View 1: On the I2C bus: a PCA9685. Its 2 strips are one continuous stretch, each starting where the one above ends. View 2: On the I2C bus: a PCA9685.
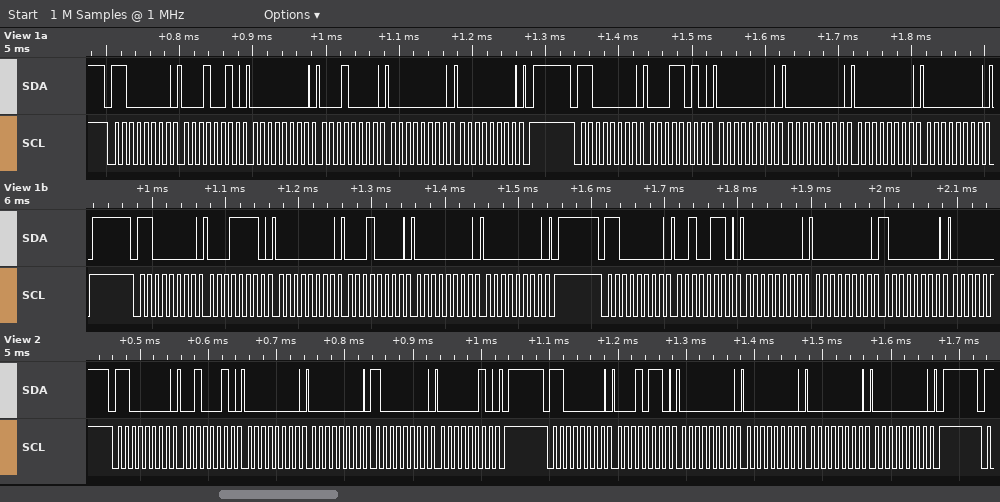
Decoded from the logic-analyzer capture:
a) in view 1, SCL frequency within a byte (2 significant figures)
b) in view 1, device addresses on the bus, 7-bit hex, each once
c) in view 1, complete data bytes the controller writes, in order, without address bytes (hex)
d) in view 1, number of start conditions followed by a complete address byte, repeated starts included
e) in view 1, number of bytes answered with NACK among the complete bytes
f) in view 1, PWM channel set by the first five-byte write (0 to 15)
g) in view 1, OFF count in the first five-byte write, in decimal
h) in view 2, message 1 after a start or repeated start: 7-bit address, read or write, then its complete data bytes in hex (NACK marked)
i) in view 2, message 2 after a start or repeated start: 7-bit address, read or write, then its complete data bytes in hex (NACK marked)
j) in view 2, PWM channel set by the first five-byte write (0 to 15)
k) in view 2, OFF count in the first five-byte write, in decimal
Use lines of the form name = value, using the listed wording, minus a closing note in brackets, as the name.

in view 1, SCL frequency within a byte = 100 kHz
in view 1, device addresses on the bus, 7-bit hex, each once = 0x60
in view 1, complete data bytes the controller writes, in order, without address bytes = 12 00 10 00 00 1A 00 00 00 00 1E 00 10 00 00 26 00 00 80
in view 1, number of start conditions followed by a complete address byte, repeated starts included = 4
in view 1, number of bytes answered with NACK among the complete bytes = 0
in view 1, PWM channel set by the first five-byte write = 3
in view 1, OFF count in the first five-byte write, in decimal = 0
in view 2, message 1 after a start or repeated start: 7-bit address, read or write, then its complete data bytes in hex = 0x60 write: 22 00 00 80 02
in view 2, message 2 after a start or repeated start: 7-bit address, read or write, then its complete data bytes in hex = 0x60 write: 16 00 00 00 00
in view 2, PWM channel set by the first five-byte write = 7
in view 2, OFF count in the first five-byte write, in decimal = 640
